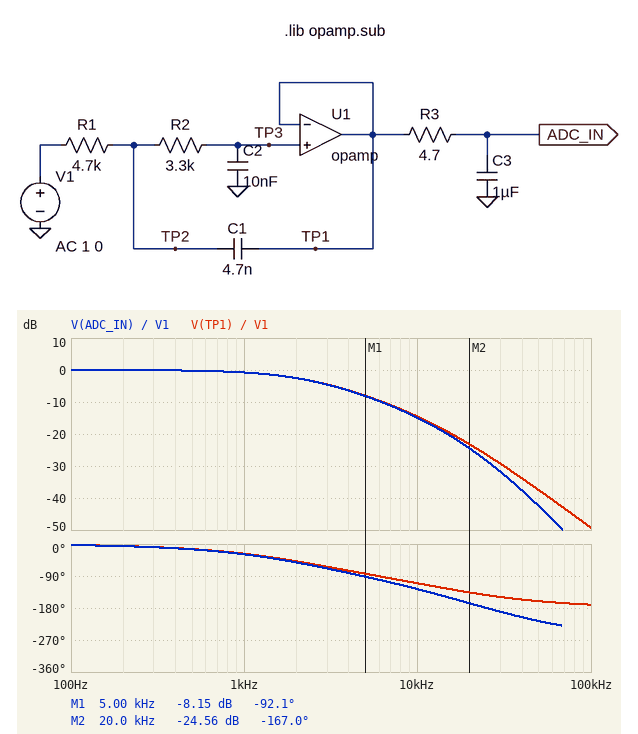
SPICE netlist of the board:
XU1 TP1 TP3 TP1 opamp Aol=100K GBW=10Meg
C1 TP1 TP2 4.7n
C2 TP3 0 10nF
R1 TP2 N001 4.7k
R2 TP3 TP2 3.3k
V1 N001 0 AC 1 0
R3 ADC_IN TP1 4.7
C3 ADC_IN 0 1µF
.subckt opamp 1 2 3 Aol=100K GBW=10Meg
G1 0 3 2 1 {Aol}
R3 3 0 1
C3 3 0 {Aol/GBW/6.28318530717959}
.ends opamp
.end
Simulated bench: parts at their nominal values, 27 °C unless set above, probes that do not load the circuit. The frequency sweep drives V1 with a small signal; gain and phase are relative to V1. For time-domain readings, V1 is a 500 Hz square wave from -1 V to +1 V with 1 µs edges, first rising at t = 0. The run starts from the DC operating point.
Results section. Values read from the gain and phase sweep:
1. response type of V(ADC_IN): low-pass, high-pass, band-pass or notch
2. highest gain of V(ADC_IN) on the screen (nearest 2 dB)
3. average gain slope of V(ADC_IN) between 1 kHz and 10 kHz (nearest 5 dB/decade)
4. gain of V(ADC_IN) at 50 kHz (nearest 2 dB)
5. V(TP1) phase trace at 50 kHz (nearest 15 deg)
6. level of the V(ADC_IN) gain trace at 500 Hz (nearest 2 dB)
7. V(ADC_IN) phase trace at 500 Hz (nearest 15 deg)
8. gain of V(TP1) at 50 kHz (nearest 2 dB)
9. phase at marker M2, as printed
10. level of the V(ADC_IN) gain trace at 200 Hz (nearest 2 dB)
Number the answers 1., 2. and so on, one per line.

1. low-pass
2. 0 dB
3. -15 dB/decade
4. -42 dB
5. -165 deg
6. 0 dB
7. -15 deg
8. -38 dB
9. -167.0 deg
10. 0 dB
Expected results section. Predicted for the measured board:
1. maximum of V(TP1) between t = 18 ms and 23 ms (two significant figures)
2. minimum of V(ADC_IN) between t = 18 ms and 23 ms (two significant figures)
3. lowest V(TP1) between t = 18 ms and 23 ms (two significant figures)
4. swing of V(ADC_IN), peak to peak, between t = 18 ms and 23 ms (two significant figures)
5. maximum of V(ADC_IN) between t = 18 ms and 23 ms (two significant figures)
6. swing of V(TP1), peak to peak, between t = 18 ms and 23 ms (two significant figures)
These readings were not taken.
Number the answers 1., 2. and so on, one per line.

1. 1.0 V
2. -1.0 V
3. -1.0 V
4. 2.0 V
5. 1.0 V
6. 2.0 V
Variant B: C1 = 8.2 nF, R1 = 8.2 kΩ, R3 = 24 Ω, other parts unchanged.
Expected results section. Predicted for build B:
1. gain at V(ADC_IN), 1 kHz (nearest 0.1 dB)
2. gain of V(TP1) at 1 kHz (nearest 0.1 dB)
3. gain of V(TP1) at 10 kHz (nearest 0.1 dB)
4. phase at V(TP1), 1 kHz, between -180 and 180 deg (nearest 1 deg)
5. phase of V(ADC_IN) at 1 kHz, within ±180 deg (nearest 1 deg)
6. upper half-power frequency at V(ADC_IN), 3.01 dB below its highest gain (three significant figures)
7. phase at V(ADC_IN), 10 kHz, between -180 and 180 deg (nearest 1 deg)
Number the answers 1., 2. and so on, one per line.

1. -1.4 dB
2. -1.3 dB
3. -20.5 dB
4. -38 deg
5. -47 deg
6. 1.56 kHz
7. 166 deg
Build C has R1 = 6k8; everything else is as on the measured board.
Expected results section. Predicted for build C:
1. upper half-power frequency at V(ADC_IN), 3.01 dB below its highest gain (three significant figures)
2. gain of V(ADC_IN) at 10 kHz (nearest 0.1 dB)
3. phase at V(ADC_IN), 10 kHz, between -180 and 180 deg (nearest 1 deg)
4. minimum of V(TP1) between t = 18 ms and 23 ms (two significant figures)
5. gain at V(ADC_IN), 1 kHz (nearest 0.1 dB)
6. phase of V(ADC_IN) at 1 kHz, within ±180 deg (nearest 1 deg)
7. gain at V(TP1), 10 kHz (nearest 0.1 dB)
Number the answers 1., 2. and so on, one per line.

1. 1.75 kHz
2. -17.4 dB
3. -133 deg
4. -1.0 V
5. -1.2 dB
6. -35 deg
7. -17.0 dB
